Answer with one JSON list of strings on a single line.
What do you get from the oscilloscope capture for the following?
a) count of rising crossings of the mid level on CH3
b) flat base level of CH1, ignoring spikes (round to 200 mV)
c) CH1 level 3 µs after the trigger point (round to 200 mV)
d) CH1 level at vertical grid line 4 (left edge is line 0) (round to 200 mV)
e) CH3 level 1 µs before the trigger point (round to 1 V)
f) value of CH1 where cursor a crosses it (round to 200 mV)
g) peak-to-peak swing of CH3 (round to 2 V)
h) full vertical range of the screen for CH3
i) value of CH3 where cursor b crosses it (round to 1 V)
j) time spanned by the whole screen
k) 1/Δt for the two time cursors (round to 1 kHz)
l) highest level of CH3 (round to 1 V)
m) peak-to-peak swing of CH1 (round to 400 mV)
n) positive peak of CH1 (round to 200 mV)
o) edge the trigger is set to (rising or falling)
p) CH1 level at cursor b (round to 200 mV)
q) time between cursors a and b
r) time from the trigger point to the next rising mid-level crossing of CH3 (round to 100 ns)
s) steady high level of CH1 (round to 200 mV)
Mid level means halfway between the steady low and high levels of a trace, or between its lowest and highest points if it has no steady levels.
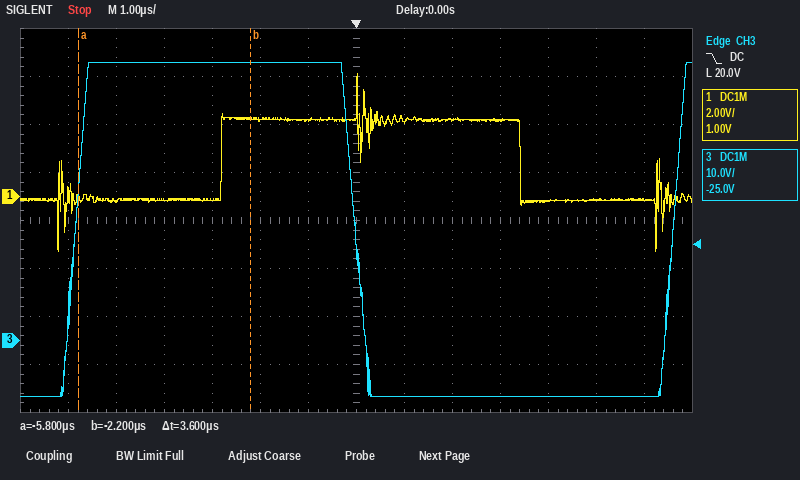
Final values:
["2", "-200 mV", "3.2 V", "-200 mV", "58 V", "-200 mV", "70 V", "80 V", "58 V", "14 µs", "278 kHz", "58 V", "7.6 V", "5.2 V", "falling", "3.2 V", "3.6 µs", "6.6 µs", "3.2 V"]
